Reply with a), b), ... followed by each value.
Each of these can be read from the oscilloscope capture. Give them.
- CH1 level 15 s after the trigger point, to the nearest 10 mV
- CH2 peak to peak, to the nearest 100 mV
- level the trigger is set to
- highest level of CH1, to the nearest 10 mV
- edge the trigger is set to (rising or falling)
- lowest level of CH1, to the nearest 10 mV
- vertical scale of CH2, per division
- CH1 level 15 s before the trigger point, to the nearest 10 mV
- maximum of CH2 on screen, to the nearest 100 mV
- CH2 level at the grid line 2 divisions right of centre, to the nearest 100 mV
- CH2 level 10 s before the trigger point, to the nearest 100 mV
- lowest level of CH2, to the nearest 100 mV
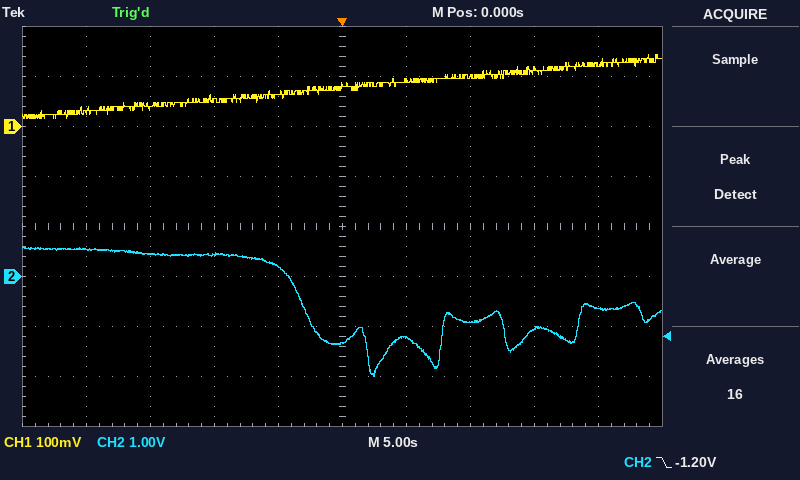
a) 110 mV
b) 2.6 V
c) -1.20 V
d) 140 mV
e) falling
f) 20 mV
g) 1 V
h) 40 mV
i) 600 mV
j) -900 mV
k) 400 mV
l) -2.0 V
